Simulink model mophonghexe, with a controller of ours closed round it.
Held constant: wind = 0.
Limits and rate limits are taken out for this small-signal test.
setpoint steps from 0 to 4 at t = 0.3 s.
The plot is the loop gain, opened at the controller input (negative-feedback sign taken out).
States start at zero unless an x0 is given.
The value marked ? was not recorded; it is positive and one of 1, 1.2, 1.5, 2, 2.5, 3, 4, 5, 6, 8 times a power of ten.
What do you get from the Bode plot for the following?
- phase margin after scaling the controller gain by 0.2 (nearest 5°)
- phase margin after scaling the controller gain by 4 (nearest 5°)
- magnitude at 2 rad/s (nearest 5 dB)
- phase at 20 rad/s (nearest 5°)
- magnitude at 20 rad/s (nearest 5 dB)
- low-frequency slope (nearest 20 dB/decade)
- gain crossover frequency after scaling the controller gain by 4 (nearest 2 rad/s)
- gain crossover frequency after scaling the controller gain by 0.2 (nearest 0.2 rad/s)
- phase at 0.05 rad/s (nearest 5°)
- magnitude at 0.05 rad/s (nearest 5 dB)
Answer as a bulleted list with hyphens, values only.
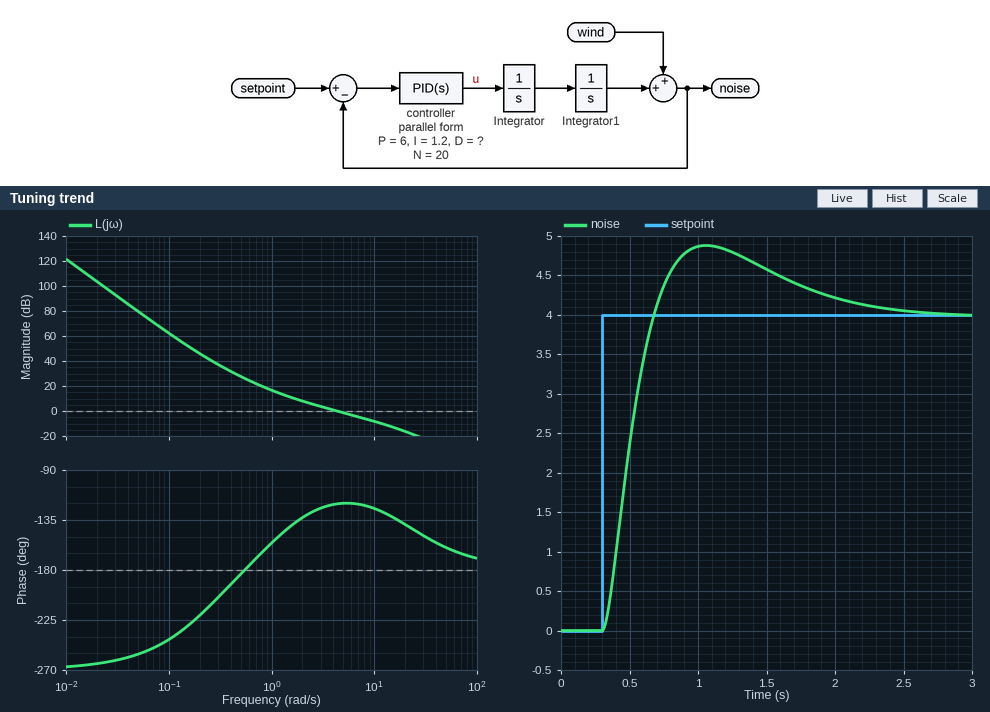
- 30°
- 50°
- 10 dB
- -140°
- -15 dB
- -60 dB/decade
- 14 rad/s
- 1.2 rad/s
- -255°
- 80 dB
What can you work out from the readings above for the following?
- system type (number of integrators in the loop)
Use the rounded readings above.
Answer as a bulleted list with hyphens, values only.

- 3
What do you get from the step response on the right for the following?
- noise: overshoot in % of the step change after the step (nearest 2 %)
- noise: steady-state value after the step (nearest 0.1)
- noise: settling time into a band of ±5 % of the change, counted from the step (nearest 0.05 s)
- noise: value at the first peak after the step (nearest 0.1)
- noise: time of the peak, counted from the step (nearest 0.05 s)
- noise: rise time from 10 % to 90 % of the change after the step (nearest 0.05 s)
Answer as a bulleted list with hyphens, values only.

- 22 %
- 4.0
- 1.75 s
- 4.9
- 0.75 s
- 0.25 s
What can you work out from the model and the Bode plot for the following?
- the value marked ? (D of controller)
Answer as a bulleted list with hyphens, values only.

- 4
